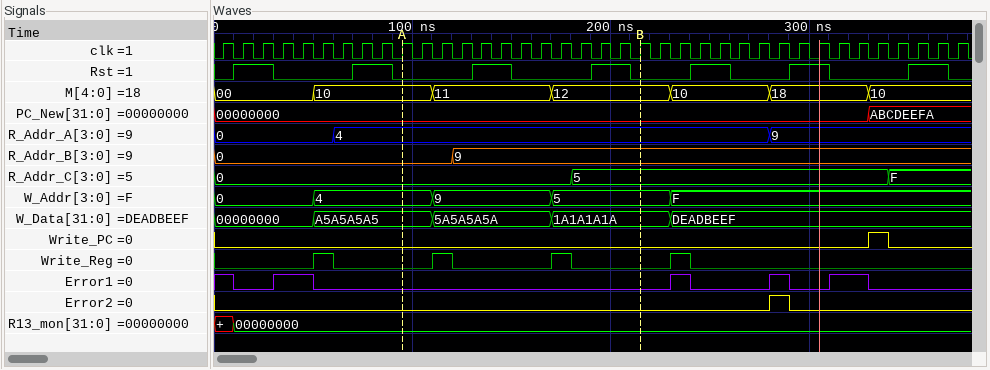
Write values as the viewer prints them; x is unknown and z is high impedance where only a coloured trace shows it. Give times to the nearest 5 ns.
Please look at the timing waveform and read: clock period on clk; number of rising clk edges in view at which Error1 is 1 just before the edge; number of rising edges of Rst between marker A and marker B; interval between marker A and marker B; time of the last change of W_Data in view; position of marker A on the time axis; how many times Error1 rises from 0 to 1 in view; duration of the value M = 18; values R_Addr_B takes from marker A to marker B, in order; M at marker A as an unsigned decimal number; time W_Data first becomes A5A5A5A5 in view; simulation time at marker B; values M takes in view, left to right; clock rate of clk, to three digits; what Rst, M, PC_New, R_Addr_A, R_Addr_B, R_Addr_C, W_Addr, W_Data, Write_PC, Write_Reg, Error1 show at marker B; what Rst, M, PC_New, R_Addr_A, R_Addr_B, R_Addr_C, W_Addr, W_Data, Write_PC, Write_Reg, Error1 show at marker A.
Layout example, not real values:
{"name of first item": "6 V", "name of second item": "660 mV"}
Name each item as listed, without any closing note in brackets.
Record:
{"clock period on clk": "10 ns", "number of rising clk edges in view at which Error1 is 1 just before the edge": "7", "number of rising edges of Rst between marker A and marker B": "2", "interval between marker A and marker B": "120 ns", "time of the last change of W_Data in view": "230 ns", "position of marker A on the time axis": "95 ns", "how many times Error1 rises from 0 to 1 in view": "4", "duration of the value M = 18": "50 ns", "values R_Addr_B takes from marker A to marker B, in order": "0, 9", "M at marker A as an unsigned decimal number": "16", "time W_Data first becomes A5A5A5A5 in view": "50 ns", "simulation time at marker B": "215 ns", "values M takes in view, left to right": "00, 10, 11, 12, 10, 18, 10", "clock rate of clk, to three digits": "100 MHz", "what Rst, M, PC_New, R_Addr_A, R_Addr_B, R_Addr_C, W_Addr, W_Data, Write_PC, Write_Reg, Error1 show at marker B": "Rst=0, M=12, PC_New=00000000, R_Addr_A=4, R_Addr_B=9, R_Addr_C=5, W_Addr=5, W_Data=1A1A1A1A, Write_PC=0, Write_Reg=0, Error1=0", "what Rst, M, PC_New, R_Addr_A, R_Addr_B, R_Addr_C, W_Addr, W_Data, Write_PC, Write_Reg, Error1 show at marker A": "Rst=0, M=10, PC_New=00000000, R_Addr_A=4, R_Addr_B=0, R_Addr_C=0, W_Addr=4, W_Data=A5A5A5A5, Write_PC=0, Write_Reg=0, Error1=0"}
